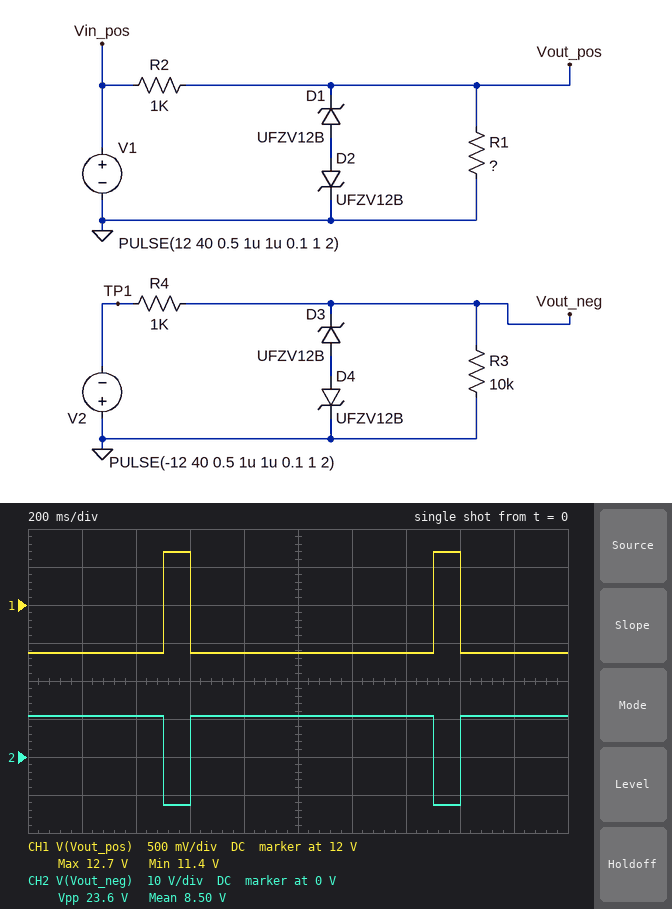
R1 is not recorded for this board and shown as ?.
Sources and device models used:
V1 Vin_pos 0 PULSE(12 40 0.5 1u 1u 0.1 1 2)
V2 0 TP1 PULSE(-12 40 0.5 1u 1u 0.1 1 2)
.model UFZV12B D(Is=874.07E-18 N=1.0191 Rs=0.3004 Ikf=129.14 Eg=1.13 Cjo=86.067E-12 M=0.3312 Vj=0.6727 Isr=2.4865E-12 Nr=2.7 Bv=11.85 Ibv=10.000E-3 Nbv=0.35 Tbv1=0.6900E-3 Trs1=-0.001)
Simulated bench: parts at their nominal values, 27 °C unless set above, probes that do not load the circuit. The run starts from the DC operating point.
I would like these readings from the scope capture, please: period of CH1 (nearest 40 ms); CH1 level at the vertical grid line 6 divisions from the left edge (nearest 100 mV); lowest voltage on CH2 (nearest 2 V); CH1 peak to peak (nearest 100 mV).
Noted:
1.00 s
11.4 V
-12 V
1.3 V
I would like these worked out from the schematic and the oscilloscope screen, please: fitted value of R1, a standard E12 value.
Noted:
18 kΩ
